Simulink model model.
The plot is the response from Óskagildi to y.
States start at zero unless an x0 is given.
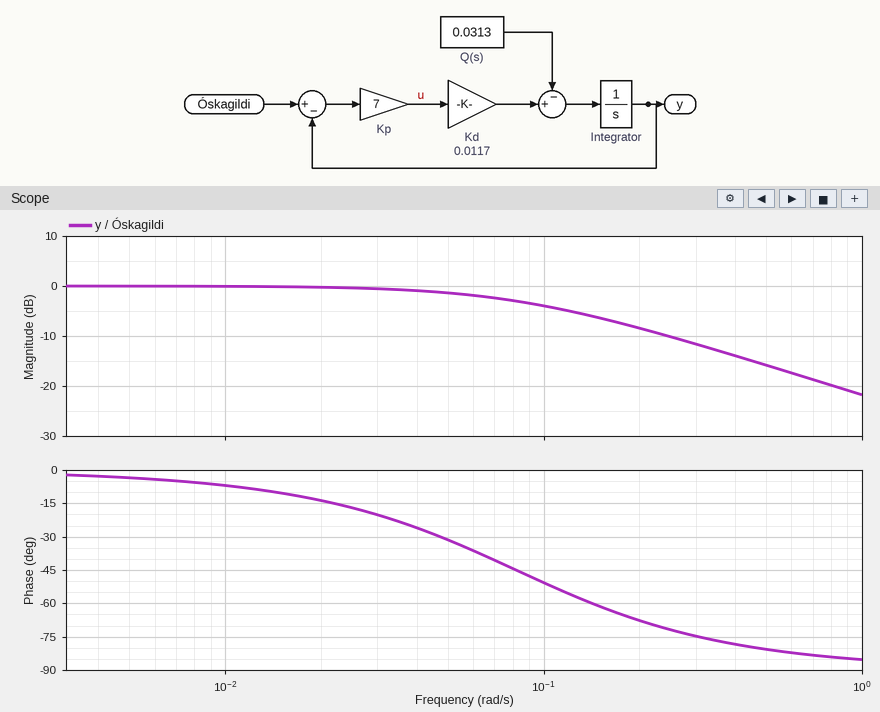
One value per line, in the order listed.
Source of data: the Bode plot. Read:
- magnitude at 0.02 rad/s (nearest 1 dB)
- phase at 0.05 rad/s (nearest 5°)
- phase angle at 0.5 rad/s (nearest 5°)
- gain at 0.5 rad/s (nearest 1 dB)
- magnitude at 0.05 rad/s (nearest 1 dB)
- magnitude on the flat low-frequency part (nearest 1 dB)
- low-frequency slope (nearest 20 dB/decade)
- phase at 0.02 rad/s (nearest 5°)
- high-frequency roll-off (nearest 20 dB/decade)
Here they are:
0 dB
-30°
-80°
-16 dB
-1 dB
0 dB
0 dB/decade
-15°
-20 dB/decade
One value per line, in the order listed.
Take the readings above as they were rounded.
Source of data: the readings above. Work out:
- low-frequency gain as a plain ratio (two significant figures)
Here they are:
1.0
